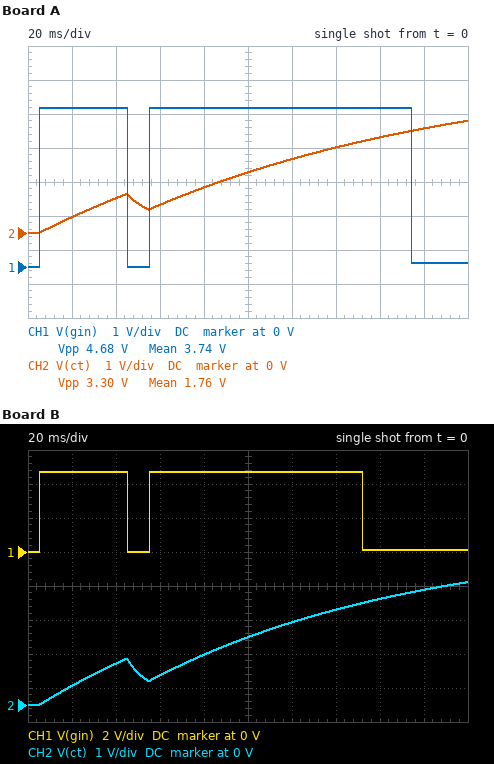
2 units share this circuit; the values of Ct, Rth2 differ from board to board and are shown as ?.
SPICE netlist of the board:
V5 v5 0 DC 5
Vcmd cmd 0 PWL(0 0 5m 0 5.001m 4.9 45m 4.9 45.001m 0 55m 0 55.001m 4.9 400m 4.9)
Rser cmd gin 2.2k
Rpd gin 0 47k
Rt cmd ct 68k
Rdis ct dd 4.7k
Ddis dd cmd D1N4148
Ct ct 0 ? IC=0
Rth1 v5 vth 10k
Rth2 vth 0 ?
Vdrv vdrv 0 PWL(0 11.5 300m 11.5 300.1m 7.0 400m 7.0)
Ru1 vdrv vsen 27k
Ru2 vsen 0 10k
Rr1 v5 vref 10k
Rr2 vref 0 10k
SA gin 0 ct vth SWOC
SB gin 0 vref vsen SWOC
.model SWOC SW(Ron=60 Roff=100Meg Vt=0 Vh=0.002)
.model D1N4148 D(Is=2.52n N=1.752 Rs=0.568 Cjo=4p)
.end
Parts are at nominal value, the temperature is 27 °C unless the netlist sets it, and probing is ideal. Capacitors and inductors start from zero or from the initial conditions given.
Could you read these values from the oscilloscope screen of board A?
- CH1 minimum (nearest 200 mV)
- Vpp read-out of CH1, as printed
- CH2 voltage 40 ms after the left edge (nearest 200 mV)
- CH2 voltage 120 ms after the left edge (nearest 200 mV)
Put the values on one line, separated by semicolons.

0 V; 4.68 V; 1.0 V; 2.2 V
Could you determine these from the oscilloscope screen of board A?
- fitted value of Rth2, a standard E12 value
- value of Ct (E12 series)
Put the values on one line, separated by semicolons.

15 kΩ; 2.2 µF
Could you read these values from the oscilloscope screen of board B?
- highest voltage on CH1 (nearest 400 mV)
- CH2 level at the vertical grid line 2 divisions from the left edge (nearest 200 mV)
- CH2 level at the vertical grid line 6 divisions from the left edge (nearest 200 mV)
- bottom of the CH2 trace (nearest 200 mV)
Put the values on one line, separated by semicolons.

4.8 V; 1.2 V; 2.4 V; 0 V
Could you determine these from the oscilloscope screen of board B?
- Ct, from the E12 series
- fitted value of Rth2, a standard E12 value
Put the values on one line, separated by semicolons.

1.8 µF; 15 kΩ
